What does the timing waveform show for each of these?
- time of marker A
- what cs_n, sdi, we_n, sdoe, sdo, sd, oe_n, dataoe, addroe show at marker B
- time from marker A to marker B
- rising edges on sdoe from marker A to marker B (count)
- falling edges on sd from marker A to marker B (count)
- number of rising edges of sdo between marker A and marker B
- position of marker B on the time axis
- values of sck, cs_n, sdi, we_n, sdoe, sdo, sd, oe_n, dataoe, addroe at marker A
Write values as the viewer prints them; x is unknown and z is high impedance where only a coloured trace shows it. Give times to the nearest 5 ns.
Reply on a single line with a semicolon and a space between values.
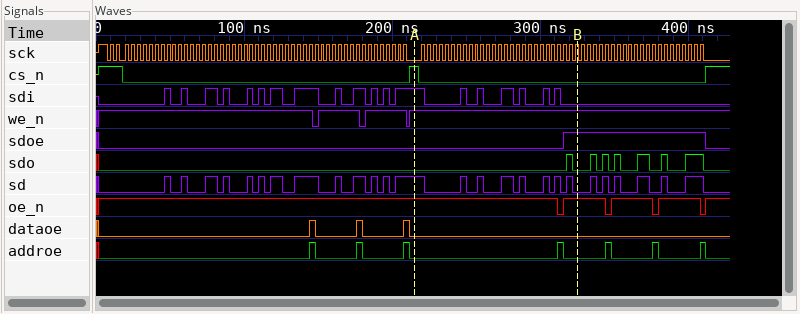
215 ns; cs_n=0, sdi=0, we_n=1, sdoe=1, sdo=0, sd=0, oe_n=1, dataoe=0, addroe=0; 110 ns; 1; 8; 1; 325 ns; sck=0, cs_n=1, sdi=1, we_n=1, sdoe=0, sdo=0, sd=1, oe_n=1, dataoe=0, addroe=0
